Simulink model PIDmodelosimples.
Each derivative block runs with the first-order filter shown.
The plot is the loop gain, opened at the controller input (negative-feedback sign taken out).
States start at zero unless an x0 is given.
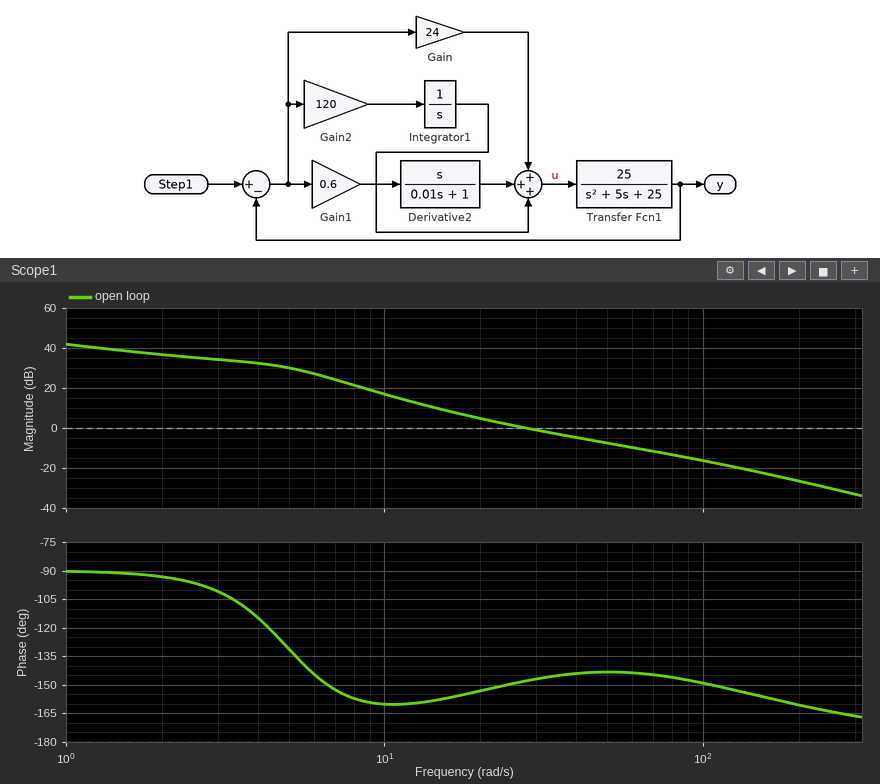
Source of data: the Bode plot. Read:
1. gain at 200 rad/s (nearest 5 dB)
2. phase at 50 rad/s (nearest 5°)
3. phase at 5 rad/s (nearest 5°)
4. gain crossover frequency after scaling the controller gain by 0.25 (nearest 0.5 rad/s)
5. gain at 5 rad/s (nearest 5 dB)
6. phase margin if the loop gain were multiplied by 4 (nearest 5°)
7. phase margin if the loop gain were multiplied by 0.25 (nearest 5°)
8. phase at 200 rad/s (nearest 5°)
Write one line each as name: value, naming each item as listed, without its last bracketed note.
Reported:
gain at 200 rad/s: -25 dB
phase at 50 rad/s: -145°
phase at 5 rad/s: -130°
gain crossover frequency after scaling the controller gain by 0.25: 13.0 rad/s
gain at 5 rad/s: 30 dB
phase margin if the loop gain were multiplied by 4: 35°
phase margin if the loop gain were multiplied by 0.25: 20°
phase at 200 rad/s: -160°
